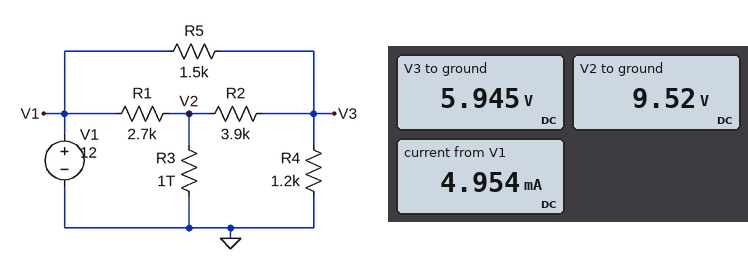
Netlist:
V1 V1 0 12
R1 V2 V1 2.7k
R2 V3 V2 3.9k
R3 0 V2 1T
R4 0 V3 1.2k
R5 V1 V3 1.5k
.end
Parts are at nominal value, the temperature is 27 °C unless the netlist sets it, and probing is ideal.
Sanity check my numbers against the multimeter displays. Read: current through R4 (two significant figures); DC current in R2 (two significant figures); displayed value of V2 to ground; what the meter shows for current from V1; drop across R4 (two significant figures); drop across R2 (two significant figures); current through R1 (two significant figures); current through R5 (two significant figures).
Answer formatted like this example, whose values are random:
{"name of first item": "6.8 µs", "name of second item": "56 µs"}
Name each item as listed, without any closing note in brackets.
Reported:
{"current through R4": "5.0 mA", "DC current in R2": "920 µA", "displayed value of V2 to ground": "9.52 V", "what the meter shows for current from V1": "4.954 mA", "drop across R4": "5.9 V", "drop across R2": "3.6 V", "current through R1": "920 µA", "current through R5": "4.0 mA"}
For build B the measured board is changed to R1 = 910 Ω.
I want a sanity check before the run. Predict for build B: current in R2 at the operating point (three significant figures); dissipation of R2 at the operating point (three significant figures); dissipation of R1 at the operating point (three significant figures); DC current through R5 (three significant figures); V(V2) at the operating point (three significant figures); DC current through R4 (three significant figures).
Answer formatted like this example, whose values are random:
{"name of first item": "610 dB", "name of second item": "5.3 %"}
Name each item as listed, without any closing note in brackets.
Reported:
{"current in R2 at the operating point": "1.22 mA", "dissipation of R2 at the operating point": "5.78 mW", "dissipation of R1 at the operating point": "1.35 mW", "DC current through R5": "3.90 mA", "V(V2) at the operating point": "10.9 V", "DC current through R4": "5.12 mA"}
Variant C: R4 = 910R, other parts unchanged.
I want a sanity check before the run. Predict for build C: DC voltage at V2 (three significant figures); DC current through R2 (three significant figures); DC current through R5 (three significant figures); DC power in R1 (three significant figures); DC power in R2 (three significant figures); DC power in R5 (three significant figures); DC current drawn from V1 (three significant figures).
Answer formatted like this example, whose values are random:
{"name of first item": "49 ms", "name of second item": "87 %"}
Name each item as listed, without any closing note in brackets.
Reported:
{"DC voltage at V2": "9.19 V", "DC current through R2": "1.04 mA", "DC current through R5": "4.59 mA", "DC power in R1": "2.93 mW", "DC power in R2": "4.24 mW", "DC power in R5": "31.5 mW", "DC current drawn from V1": "5.63 mA"}
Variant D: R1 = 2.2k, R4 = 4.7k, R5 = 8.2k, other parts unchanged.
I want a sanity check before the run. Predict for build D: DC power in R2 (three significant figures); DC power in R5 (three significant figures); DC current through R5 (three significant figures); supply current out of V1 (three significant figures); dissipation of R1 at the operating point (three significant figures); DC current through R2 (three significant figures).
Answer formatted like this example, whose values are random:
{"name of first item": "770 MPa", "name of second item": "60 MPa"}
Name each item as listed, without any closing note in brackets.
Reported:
{"DC power in R2": "2.75 mW", "DC power in R5": "3.20 mW", "DC current through R5": "624 µA", "supply current out of V1": "1.46 mA", "dissipation of R1 at the operating point": "1.55 mW", "DC current through R2": "839 µA"}
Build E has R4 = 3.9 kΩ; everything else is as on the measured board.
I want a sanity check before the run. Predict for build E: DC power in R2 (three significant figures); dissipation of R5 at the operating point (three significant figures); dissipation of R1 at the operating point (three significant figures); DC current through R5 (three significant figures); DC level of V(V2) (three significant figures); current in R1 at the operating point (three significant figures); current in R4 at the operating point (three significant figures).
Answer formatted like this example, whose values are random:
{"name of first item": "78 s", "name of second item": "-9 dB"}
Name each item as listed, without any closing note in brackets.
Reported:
{"DC power in R2": "734 µW", "dissipation of R5 at the operating point": "5.47 mW", "dissipation of R1 at the operating point": "508 µW", "DC current through R5": "1.91 mA", "DC level of V(V2)": "10.8 V", "current in R1 at the operating point": "434 µA", "current in R4 at the operating point": "2.34 mA"}
